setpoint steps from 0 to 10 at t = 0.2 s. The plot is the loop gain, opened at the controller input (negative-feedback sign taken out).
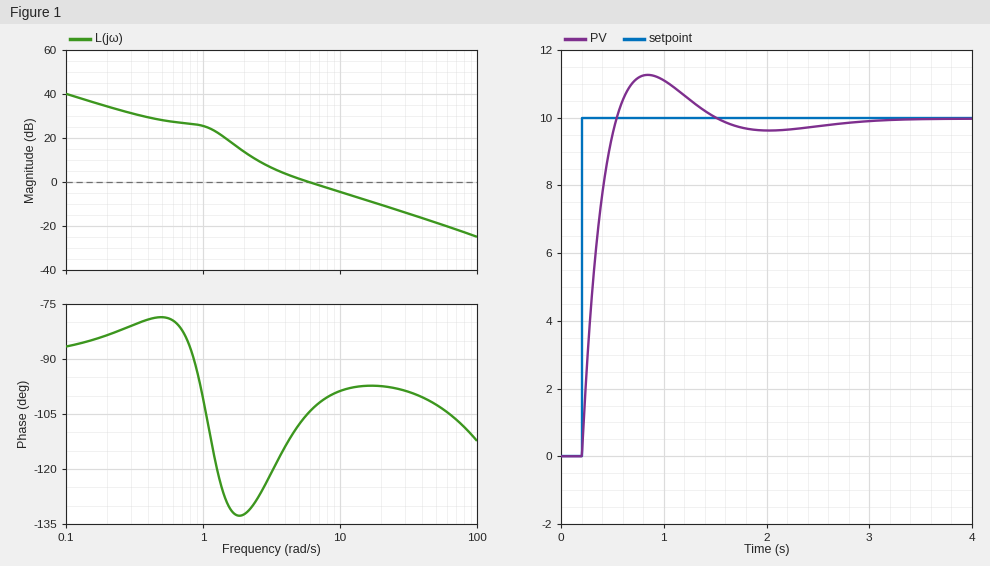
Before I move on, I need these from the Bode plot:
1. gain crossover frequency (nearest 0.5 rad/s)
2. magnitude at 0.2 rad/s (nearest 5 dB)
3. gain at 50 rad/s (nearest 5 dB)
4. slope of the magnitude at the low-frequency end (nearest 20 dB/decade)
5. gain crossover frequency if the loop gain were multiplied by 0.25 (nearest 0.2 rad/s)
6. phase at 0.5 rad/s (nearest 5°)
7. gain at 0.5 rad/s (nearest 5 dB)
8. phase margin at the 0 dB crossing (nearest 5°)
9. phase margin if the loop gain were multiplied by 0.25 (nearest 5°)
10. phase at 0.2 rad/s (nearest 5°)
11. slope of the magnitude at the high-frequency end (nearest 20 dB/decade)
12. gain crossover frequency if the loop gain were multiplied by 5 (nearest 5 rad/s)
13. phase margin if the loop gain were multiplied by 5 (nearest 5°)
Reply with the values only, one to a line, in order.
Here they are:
6.0 rad/s
35 dB
-20 dB
-20 dB/decade
2.2 rad/s
-80°
30 dB
75°
50°
-85°
-20 dB/decade
30 rad/s
80°
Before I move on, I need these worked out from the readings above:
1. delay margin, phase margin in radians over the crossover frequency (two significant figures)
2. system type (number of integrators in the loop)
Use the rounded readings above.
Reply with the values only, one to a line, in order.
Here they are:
0.22 s
1
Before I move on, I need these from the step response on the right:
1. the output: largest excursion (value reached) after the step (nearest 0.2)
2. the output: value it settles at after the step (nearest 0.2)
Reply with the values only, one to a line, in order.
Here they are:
11.2
10.0
